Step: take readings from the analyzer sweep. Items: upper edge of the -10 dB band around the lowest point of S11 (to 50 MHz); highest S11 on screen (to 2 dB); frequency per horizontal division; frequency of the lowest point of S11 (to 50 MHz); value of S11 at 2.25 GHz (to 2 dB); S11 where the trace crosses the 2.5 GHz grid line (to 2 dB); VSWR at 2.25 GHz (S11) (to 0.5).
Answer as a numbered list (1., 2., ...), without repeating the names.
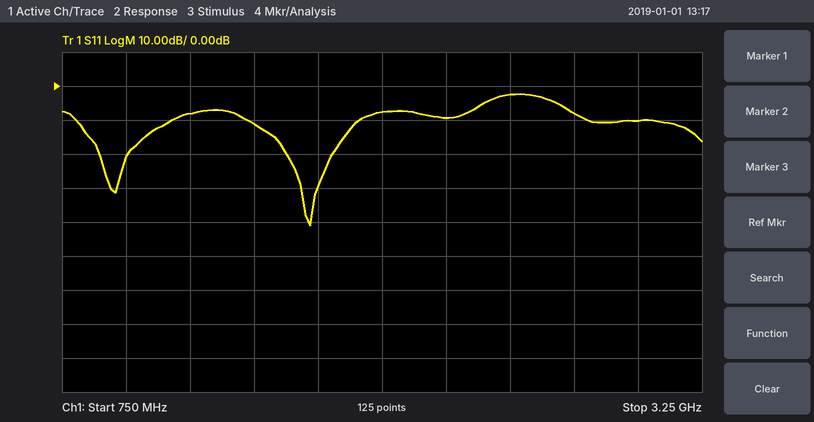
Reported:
1. 1.90 GHz
2. -2 dB
3. 250 MHz
4. 1.70 GHz
5. -10 dB
6. -2 dB
7. 2.0
